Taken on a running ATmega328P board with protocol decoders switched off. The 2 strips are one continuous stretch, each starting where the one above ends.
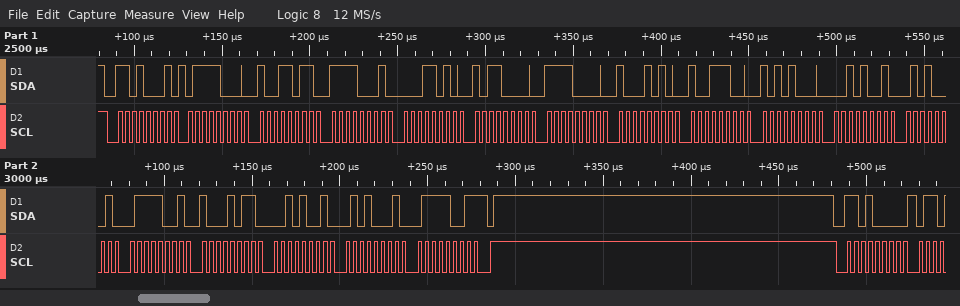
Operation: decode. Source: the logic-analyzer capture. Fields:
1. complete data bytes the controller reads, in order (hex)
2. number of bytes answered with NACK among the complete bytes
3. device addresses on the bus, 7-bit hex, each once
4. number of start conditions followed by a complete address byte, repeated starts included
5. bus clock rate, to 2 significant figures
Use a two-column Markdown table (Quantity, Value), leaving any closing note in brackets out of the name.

| Quantity | Value |
|---|---|
| complete data bytes the controller reads, in order | 78 9B F1 1A B0 F0 8A 9C A8 29 51 79 8B 29 51 79 |
| number of bytes answered with NACK among the complete bytes | 1 |
| device addresses on the bus, 7-bit hex, each once | 0x68 |
| number of start conditions followed by a complete address byte, repeated starts included | 2 |
| bus clock rate, to 2 significant figures | 250 kHz |
